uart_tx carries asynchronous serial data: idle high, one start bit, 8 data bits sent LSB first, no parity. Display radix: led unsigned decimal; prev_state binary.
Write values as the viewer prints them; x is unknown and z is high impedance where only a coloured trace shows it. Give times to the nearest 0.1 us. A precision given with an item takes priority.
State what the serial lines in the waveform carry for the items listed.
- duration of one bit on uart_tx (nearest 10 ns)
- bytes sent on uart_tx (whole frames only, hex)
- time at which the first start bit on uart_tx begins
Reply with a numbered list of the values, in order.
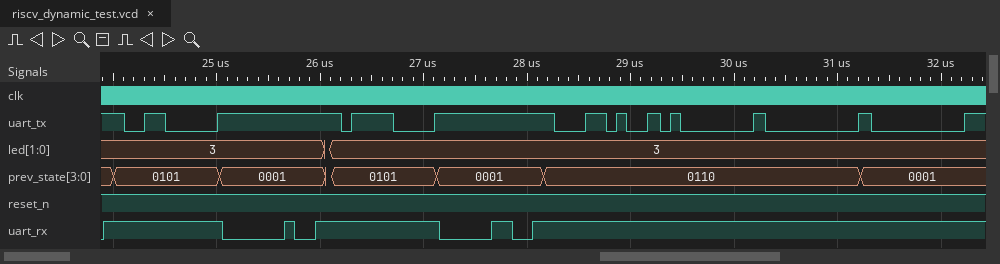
1. 100 ns
2. 06, 0F, 2C, 01, 00, 00
3. 24.1 us
